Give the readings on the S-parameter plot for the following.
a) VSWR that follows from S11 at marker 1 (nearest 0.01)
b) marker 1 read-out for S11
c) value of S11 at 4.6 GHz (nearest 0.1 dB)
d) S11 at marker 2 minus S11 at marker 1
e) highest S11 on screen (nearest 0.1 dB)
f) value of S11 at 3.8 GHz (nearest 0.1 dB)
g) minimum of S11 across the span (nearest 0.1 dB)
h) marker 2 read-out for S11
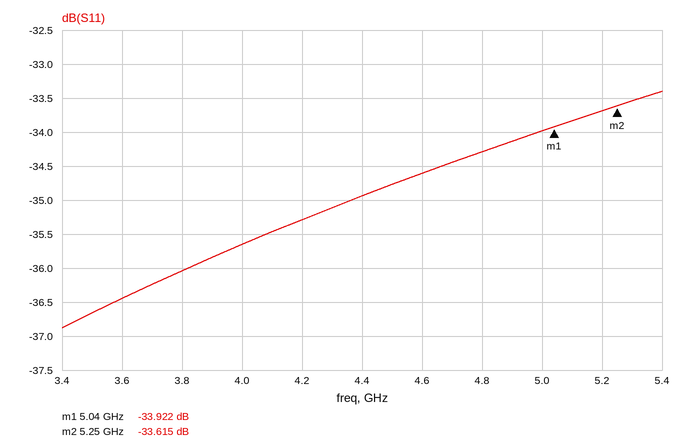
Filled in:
1.04
-33.922 dB
-34.6 dB
0.307 dB
-33.4 dB
-36.0 dB
-36.9 dB
-33.615 dB
